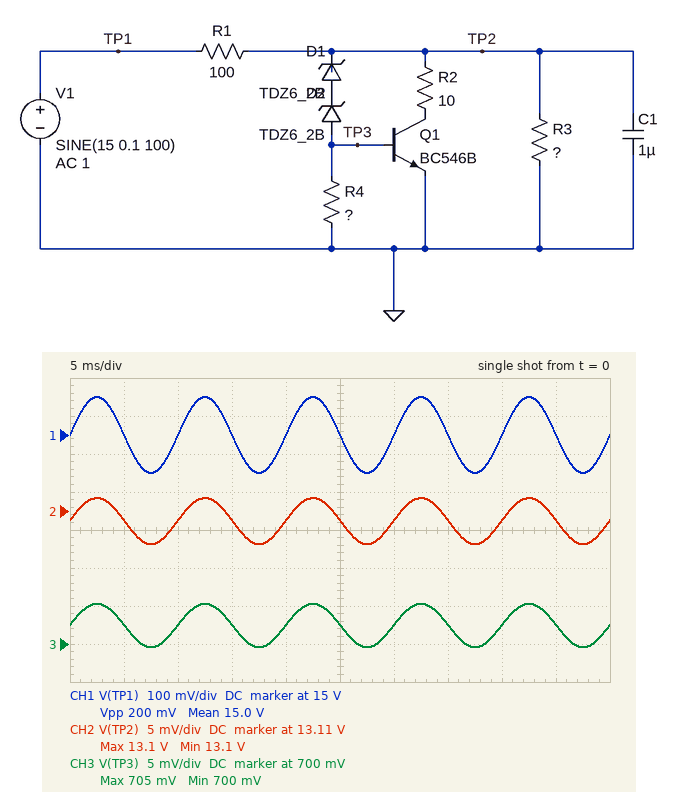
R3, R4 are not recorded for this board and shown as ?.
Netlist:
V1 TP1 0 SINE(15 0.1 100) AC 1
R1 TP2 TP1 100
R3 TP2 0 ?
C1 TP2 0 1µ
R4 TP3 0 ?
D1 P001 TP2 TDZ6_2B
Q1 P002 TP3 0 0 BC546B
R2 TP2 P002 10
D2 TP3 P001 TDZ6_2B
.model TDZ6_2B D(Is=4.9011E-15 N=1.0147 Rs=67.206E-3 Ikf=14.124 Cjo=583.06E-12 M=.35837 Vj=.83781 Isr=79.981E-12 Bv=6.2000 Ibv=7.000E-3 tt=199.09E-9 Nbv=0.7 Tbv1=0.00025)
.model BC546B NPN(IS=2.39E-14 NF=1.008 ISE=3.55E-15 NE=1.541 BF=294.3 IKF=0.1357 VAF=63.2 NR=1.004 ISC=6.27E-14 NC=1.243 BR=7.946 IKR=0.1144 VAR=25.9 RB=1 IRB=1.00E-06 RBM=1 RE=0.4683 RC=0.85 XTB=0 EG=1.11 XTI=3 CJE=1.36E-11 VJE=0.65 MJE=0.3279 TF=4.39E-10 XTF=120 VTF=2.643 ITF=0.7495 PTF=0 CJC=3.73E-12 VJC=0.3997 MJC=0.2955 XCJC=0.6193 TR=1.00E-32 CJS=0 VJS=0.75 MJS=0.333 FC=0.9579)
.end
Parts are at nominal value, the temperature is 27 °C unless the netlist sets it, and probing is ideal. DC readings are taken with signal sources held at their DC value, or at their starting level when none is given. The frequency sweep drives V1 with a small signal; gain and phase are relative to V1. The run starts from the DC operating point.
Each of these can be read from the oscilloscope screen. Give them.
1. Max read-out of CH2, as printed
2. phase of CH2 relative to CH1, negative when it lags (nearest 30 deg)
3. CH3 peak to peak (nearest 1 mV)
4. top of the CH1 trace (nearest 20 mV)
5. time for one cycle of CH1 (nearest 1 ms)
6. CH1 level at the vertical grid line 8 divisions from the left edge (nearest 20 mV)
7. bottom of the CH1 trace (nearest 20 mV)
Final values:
13.1 V
0 deg
6 mV
15.10 V
10 ms
15.00 V
14.90 V
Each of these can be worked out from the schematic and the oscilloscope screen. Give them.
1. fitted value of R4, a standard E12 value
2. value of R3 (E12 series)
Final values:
100 Ω
12 kΩ
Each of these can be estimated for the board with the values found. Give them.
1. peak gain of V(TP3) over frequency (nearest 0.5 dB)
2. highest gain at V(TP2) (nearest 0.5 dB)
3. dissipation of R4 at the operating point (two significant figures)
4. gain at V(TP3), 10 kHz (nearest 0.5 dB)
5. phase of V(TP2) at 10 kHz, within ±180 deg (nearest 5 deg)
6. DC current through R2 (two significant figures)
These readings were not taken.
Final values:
-31.0 dB
-30.5 dB
4.9 mW
-31.0 dB
-10 deg
11 mA
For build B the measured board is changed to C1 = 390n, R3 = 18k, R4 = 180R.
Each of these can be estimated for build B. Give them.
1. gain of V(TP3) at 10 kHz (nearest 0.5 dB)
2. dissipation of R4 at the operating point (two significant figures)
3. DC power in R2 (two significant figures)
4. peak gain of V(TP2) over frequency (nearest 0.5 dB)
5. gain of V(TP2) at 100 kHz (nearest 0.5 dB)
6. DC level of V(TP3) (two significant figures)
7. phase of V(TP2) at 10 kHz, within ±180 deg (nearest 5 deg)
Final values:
-32.5 dB
2.8 mW
2.1 mW
-32.0 dB
-33.5 dB
710 mV
-5 deg
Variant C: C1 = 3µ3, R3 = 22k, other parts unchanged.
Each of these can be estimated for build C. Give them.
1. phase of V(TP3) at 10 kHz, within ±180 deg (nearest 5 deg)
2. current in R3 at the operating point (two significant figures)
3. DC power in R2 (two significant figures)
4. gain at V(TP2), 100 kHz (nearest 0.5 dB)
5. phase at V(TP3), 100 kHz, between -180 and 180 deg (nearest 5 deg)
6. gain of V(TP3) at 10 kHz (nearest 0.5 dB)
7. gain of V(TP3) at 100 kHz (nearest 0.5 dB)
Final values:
-30 deg
600 µA
1.3 mW
-46.5 dB
-80 deg
-32.5 dB
-47.0 dB
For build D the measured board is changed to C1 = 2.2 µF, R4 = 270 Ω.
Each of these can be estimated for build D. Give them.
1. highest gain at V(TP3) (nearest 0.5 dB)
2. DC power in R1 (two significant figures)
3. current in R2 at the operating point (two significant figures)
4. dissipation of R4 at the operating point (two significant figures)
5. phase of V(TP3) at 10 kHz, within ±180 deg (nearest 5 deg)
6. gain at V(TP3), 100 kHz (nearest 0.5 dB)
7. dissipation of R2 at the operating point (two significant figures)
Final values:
-33.0 dB
37 mW
15 mA
1.9 mW
-20 deg
-44.0 dB
2.4 mW
